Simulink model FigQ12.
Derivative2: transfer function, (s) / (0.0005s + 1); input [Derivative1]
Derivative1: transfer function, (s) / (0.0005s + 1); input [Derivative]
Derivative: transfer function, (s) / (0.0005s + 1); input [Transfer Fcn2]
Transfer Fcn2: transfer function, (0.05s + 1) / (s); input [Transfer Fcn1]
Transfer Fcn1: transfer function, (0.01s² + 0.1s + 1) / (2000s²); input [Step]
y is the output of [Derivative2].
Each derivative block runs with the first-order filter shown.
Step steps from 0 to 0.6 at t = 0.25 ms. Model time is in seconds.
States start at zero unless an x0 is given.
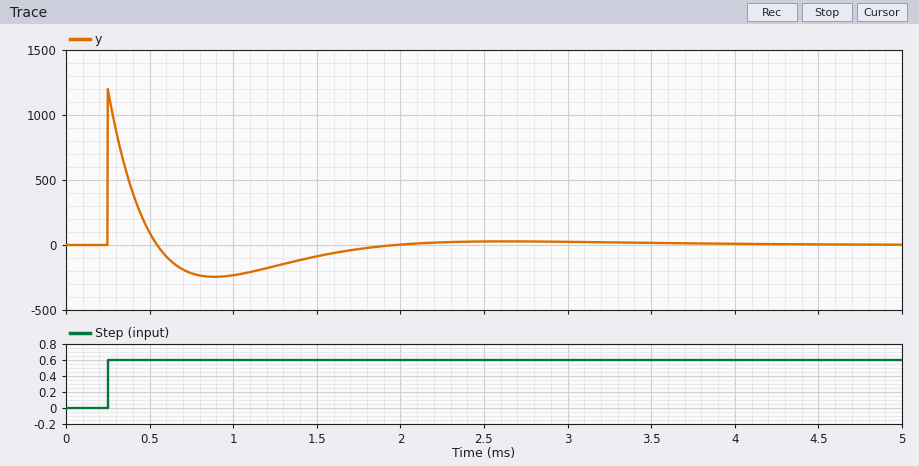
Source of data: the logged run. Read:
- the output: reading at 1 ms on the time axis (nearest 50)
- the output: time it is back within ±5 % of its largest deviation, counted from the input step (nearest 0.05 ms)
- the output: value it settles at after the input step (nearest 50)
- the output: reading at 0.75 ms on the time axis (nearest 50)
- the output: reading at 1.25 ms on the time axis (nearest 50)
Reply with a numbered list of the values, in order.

1. -250
2. 1.35 ms
3. 0
4. -200
5. -150
